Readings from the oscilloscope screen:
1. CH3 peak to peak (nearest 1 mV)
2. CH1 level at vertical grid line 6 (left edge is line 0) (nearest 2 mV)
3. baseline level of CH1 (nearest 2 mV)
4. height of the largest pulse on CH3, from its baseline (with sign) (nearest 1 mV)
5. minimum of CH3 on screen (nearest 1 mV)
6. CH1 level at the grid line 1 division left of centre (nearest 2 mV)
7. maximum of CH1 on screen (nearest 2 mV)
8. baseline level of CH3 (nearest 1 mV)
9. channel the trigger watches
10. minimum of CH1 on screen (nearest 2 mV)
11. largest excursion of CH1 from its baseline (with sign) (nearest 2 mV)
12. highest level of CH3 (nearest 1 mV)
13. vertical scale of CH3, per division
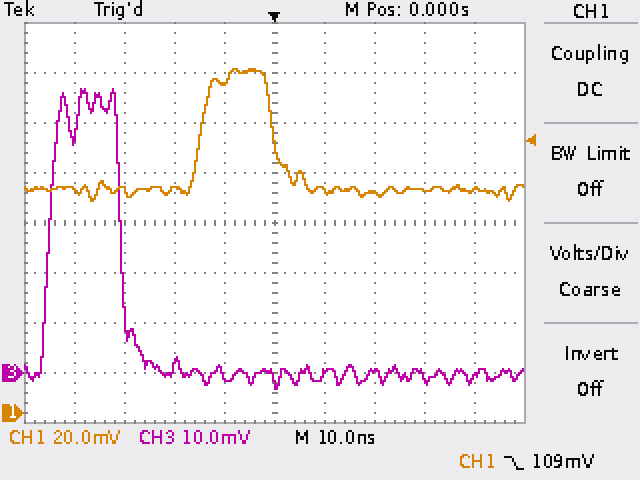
60 mV
88 mV
90 mV
+57 mV
-3 mV
132 mV
138 mV
0 mV
CH1
84 mV
+48 mV
57 mV
10 mV
